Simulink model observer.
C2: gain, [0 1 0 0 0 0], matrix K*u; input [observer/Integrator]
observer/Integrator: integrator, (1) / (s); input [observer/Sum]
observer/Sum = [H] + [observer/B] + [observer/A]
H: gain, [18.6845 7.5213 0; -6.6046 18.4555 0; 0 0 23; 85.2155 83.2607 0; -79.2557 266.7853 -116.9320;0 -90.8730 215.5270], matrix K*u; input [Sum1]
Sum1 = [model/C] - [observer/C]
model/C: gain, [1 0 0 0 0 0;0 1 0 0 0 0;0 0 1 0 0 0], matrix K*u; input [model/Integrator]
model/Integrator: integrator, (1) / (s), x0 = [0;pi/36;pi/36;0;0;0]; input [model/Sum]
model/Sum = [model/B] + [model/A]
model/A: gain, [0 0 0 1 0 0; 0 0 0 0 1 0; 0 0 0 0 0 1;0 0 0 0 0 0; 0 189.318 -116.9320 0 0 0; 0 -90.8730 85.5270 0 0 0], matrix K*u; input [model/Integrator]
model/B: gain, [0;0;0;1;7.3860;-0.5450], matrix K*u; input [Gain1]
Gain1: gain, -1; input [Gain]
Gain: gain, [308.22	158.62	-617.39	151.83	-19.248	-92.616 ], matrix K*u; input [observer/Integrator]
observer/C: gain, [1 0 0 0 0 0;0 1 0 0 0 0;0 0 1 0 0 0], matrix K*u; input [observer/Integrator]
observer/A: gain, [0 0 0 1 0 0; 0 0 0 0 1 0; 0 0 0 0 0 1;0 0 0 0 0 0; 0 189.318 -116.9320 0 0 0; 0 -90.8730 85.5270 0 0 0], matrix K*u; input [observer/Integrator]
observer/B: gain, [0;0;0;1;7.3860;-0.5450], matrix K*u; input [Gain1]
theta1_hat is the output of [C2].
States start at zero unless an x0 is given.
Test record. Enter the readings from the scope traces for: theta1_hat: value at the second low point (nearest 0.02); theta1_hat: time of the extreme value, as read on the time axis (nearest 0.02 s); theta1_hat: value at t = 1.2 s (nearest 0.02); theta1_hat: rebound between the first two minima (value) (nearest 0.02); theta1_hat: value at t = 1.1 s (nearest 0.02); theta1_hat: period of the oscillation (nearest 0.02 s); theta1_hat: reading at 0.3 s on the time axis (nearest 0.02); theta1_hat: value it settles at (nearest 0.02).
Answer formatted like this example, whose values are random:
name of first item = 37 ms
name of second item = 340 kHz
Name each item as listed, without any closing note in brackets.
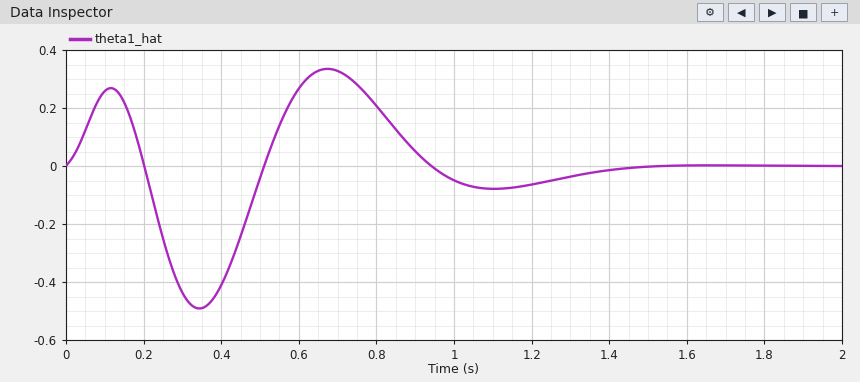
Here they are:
theta1_hat: value at the second low point = -0.08
theta1_hat: time of the extreme value, as read on the time axis = 0.34 s
theta1_hat: value at t = 1.2 s = -0.06
theta1_hat: rebound between the first two minima (value) = 0.34
theta1_hat: value at t = 1.1 s = -0.08
theta1_hat: period of the oscillation = 0.76 s
theta1_hat: reading at 0.3 s on the time axis = -0.44
theta1_hat: value it settles at = 0.00
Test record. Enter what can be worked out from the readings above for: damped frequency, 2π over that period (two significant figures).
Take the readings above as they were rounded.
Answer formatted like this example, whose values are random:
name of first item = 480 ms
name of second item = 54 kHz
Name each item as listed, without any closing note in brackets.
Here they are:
damped frequency, 2π over that period = 8.3 rad/s
